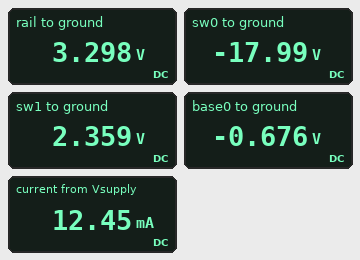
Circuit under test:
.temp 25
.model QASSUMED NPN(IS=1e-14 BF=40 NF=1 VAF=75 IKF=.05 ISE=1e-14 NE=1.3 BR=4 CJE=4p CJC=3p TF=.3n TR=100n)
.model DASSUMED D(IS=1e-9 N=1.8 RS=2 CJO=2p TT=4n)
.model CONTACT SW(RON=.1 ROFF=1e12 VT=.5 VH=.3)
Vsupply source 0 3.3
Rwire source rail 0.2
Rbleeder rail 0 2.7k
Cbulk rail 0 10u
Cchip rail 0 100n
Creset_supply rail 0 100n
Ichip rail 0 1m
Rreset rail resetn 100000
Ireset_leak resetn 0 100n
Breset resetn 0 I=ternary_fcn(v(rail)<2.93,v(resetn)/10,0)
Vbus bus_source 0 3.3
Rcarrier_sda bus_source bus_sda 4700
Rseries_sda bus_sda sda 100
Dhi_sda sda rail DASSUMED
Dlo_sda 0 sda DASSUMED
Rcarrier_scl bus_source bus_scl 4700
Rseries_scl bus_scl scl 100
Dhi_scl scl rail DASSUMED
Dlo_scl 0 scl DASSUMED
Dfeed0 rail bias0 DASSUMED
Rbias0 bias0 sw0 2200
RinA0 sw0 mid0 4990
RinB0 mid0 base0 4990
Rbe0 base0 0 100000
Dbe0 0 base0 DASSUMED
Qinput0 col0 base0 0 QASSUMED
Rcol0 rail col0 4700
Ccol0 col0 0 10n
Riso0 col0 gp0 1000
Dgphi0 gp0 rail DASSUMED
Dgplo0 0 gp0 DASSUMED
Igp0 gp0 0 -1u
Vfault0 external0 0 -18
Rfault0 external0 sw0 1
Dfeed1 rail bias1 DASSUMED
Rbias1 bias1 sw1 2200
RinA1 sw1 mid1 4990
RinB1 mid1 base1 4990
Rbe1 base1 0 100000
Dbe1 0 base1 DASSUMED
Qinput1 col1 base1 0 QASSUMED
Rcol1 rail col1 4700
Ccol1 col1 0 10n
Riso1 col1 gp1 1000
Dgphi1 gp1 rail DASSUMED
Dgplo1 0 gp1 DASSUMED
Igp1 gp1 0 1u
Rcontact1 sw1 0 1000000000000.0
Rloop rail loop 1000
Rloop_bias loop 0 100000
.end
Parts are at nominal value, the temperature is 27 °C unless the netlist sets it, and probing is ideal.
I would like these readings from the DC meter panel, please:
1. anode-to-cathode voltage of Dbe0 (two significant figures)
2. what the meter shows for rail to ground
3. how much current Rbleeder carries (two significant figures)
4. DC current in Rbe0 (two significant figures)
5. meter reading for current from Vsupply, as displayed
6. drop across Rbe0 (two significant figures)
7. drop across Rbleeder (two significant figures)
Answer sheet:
680 mV
3.298 V
1.2 mA
6.8 µA
12.45 mA
680 mV
3.3 V
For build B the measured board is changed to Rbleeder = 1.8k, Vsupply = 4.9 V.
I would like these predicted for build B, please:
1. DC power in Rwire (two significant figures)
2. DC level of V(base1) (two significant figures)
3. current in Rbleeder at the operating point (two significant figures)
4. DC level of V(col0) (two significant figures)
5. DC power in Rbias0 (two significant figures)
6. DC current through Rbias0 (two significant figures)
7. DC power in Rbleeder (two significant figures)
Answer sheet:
46 µW
680 mV
2.7 mA
4.9 V
220 mW
10 mA
13 mW
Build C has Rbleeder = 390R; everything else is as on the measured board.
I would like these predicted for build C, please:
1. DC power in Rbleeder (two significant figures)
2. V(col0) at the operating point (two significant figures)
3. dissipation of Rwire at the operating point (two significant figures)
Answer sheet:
28 mW
3.3 V
77 µW
